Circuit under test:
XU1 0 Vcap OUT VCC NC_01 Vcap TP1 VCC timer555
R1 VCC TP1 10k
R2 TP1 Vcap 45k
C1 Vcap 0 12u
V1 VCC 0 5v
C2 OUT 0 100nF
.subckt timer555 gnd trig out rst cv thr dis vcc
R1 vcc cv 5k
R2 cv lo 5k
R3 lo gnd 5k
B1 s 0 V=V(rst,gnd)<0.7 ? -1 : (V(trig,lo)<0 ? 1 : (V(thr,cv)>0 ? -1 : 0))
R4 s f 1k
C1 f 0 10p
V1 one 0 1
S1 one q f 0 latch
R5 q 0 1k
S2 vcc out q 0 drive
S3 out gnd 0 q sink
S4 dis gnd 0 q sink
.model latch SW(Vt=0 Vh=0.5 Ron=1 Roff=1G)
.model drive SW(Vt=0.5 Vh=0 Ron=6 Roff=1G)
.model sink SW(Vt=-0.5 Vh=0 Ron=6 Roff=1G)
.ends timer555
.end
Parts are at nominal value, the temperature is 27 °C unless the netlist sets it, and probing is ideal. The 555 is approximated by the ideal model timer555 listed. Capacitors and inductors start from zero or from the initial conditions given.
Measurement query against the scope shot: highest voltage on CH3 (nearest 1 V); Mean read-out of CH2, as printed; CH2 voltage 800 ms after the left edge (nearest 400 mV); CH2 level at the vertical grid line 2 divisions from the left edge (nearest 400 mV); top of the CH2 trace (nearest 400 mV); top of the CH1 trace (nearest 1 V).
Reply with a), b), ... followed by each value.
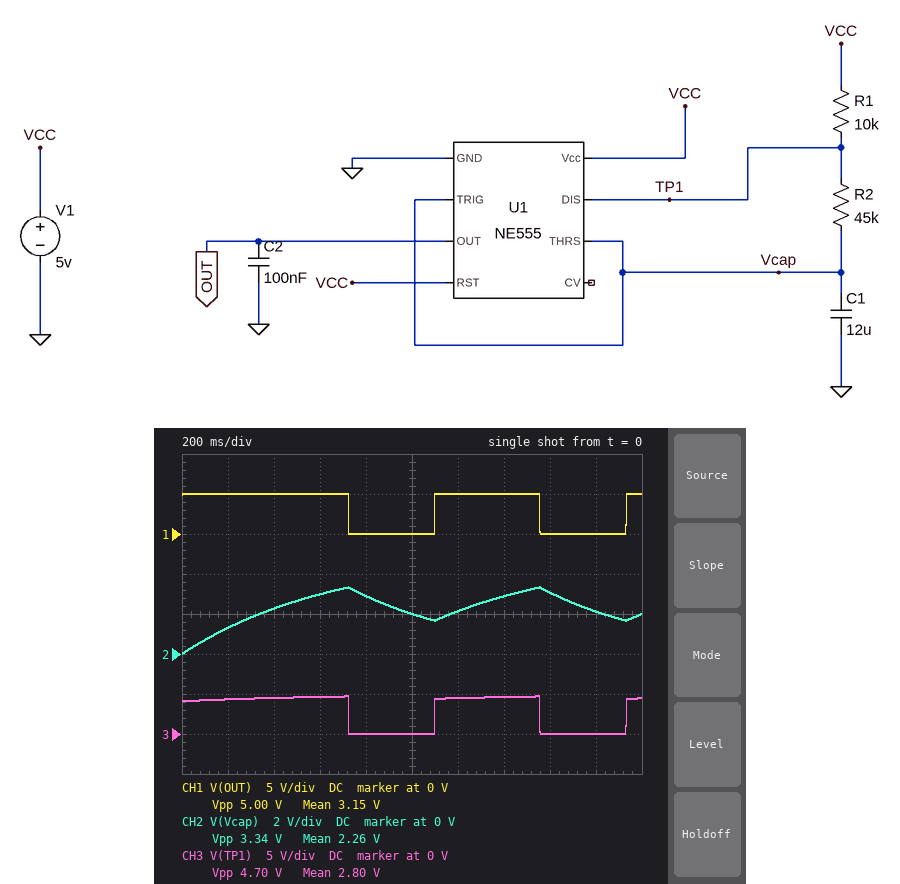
a) 5 V
b) 2.26 V
c) 2.8 V
d) 2.4 V
e) 3.2 V
f) 5 V
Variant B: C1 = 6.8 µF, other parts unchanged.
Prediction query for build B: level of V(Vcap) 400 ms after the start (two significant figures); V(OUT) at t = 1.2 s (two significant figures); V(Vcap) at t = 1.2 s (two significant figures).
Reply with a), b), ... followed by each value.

a) 3.3 V
b) 5.0 V
c) 2.5 V
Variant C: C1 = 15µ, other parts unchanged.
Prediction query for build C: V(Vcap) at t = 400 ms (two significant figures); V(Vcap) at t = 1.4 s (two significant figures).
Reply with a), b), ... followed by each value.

a) 1.9 V
b) 1.8 V
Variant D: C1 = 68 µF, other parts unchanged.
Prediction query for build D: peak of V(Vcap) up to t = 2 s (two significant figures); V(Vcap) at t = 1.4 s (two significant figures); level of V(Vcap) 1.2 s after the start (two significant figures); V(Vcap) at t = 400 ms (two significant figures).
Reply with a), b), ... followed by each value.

a) 2.1 V
b) 1.6 V
c) 1.4 V
d) 510 mV
